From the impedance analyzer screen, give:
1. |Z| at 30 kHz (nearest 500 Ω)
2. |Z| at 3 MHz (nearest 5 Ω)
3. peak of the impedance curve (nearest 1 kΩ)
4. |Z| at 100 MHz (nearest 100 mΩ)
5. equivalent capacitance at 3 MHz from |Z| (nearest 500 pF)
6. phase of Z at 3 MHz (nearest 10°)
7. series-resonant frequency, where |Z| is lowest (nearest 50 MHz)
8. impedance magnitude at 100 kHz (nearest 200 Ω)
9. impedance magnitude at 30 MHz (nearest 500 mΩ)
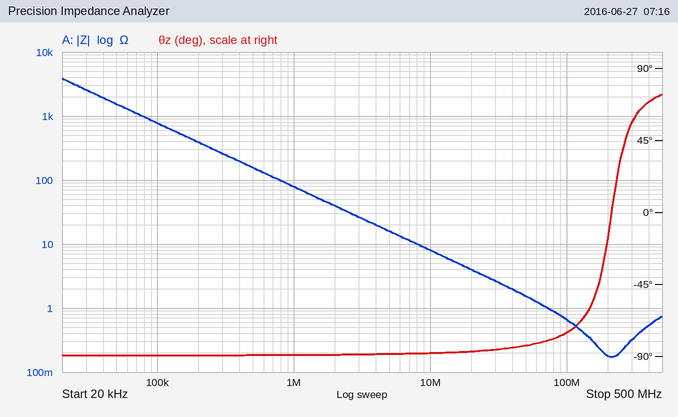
2.5 kΩ
25 Ω
4 kΩ
700 mΩ
2.0 nF
-90°
200 MHz
800 Ω
2.5 Ω
